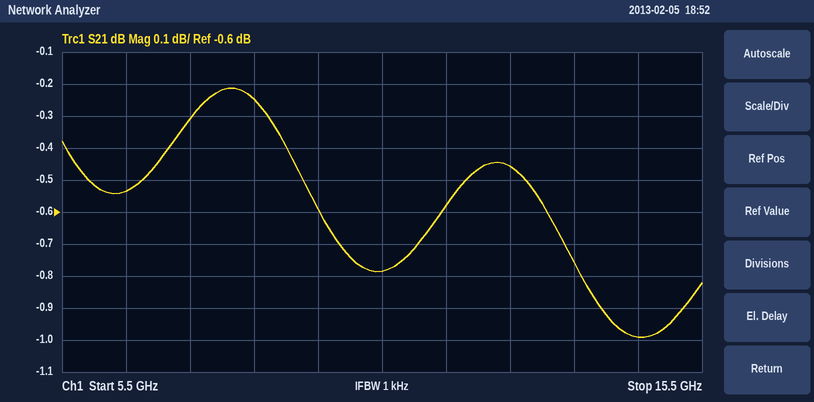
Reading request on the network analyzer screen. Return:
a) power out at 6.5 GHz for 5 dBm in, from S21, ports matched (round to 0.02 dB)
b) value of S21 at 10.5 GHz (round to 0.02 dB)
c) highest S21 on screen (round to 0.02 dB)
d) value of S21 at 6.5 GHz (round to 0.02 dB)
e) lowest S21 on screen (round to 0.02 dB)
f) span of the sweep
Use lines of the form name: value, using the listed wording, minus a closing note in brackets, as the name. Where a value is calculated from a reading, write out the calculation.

power out at 6.5 GHz for 5 dBm in, from S21, ports matched: 5 dBm + (-0.54 dB) = 4.46 dBm
value of S21 at 10.5 GHz: -0.78 dB
highest S21 on screen: -0.22 dB
value of S21 at 6.5 GHz: -0.54 dB
lowest S21 on screen: -1.00 dB
span of the sweep: 10 GHz
